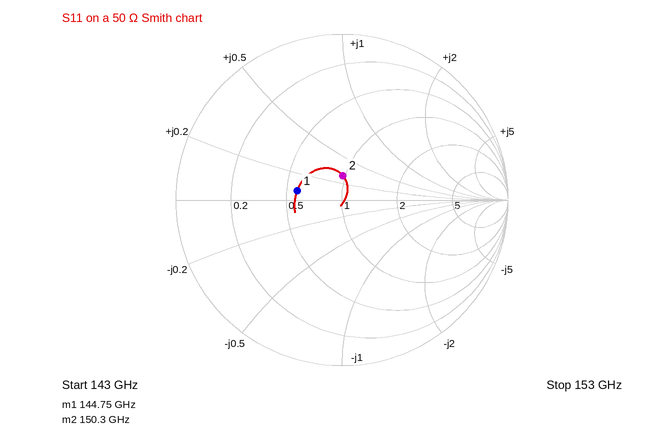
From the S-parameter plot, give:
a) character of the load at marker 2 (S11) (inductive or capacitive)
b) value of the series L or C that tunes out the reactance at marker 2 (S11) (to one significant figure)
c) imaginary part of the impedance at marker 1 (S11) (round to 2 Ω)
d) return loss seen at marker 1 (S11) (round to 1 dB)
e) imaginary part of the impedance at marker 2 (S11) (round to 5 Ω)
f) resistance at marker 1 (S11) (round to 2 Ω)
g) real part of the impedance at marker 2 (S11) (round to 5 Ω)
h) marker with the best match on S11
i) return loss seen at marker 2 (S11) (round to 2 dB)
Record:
inductive
70 fF
+4 Ω
11 dB
+15 Ω
28 Ω
50 Ω
marker 2
16 dB
